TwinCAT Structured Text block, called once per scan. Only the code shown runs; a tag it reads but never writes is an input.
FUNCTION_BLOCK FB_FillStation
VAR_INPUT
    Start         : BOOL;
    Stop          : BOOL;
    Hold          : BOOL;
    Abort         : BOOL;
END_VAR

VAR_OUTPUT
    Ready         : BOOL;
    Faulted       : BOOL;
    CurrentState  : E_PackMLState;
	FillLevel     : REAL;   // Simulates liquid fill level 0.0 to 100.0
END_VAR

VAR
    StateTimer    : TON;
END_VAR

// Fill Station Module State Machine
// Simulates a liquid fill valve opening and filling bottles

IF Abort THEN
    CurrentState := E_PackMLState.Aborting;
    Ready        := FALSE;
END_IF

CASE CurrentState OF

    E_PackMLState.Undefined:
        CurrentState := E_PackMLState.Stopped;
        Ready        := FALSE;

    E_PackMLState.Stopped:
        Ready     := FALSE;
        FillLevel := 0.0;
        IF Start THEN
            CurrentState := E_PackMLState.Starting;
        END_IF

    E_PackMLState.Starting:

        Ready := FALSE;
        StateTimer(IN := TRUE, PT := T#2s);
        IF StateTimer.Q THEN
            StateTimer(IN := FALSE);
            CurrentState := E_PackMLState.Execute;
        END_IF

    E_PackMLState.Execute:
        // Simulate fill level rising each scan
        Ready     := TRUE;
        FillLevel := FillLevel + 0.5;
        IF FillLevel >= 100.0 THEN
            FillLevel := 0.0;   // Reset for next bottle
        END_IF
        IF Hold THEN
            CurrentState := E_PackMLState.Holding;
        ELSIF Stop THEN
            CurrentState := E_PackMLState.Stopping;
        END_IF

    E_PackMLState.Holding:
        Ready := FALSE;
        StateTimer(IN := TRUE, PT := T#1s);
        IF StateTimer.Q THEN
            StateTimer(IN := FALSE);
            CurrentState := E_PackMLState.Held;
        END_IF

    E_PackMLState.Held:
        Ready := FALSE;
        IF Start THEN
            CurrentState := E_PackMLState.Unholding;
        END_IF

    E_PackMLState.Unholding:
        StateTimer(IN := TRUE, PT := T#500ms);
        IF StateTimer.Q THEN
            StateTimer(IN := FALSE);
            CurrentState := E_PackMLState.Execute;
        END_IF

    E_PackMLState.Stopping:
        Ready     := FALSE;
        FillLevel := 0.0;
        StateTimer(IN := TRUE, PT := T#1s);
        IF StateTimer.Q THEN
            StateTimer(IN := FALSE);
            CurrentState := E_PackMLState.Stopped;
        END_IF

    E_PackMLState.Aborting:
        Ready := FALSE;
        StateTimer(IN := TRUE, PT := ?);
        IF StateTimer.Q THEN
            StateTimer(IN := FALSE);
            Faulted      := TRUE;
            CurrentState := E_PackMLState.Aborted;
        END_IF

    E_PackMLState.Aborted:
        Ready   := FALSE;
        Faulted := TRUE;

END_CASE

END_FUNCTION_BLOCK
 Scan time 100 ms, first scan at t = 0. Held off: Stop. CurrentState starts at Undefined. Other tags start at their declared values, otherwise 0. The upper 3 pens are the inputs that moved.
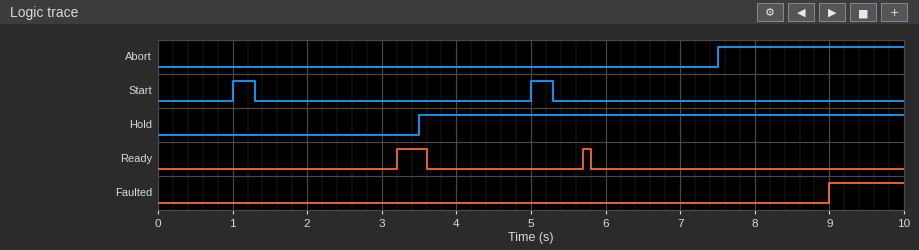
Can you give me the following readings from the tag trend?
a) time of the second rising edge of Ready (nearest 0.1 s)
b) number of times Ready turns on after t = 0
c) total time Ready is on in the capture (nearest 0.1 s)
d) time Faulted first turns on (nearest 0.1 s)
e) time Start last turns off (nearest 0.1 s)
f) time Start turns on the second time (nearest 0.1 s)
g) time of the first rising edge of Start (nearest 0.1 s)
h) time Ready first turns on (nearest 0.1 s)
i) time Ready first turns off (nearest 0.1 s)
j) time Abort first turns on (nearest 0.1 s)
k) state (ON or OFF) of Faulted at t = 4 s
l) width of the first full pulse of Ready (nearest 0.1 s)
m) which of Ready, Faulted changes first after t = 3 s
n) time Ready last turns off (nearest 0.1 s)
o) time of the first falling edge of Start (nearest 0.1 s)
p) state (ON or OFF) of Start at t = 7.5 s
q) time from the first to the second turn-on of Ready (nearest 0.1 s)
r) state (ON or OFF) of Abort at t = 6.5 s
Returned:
5.7 s
2
0.5 s
9.0 s
5.3 s
5.0 s
1.0 s
3.2 s
3.6 s
7.5 s
OFF
0.4 s
Ready
5.8 s
1.3 s
OFF
2.5 s
OFF
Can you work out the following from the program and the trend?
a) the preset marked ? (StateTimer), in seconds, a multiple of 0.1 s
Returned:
1.5 s
